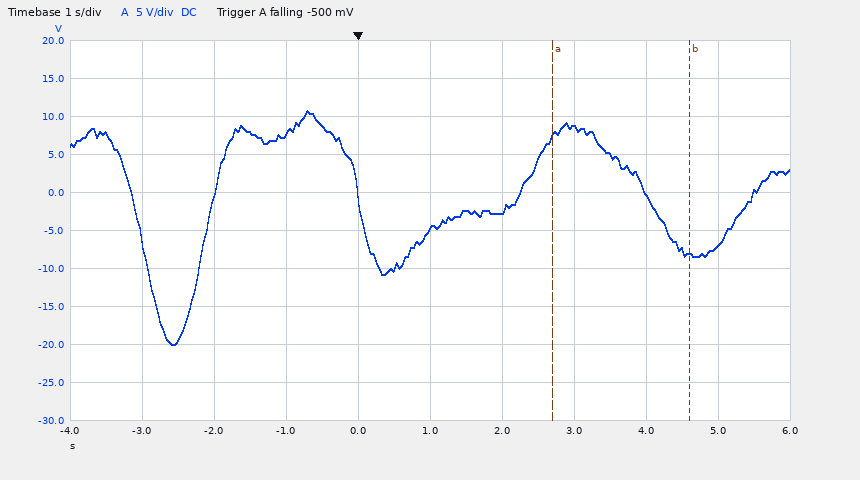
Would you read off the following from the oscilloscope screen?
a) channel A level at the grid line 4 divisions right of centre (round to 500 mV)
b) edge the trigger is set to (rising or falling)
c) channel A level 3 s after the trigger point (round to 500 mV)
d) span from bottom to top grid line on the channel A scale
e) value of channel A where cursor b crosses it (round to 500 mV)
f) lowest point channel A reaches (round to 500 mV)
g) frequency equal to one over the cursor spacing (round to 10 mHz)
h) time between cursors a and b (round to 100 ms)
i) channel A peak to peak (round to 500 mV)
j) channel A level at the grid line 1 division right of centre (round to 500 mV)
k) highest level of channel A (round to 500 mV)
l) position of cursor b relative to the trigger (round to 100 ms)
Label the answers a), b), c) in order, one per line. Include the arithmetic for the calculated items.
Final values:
a) -7.0 V
b) falling
c) 8.5 V
d) 50 V
e) -8.0 V
f) -20.0 V
g) 1 / 1.9 s ≈ 530 mHz
h) 1.9 s
i) 11.0 V − (-20.0 V) = 31.0 V
j) -2.5 V
k) 11.0 V
l) +4.6 s
